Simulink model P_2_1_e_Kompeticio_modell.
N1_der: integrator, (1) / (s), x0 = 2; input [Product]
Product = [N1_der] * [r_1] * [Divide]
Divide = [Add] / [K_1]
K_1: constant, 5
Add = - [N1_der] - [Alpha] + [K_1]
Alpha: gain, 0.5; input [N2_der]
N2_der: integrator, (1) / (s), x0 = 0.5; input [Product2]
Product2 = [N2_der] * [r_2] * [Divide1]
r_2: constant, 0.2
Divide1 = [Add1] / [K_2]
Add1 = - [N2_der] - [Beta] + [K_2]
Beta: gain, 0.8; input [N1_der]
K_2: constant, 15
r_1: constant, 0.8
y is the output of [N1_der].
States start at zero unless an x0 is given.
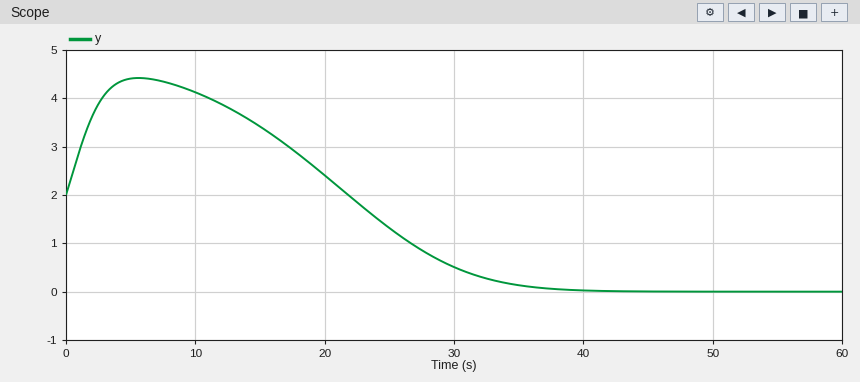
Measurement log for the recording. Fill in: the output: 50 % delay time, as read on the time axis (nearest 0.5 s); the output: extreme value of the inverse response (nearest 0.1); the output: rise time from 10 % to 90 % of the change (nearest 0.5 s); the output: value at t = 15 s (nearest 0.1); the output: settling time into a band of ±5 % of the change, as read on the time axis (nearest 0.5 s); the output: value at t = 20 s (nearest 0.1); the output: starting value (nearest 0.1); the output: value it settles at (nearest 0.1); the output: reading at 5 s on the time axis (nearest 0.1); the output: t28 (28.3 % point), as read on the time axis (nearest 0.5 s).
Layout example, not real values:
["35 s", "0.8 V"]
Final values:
["26.5 s", "4.4", "11.0 s", "3.4", "36.0 s", "2.4", "2.0", "0.0", "4.4", "24.5 s"]
